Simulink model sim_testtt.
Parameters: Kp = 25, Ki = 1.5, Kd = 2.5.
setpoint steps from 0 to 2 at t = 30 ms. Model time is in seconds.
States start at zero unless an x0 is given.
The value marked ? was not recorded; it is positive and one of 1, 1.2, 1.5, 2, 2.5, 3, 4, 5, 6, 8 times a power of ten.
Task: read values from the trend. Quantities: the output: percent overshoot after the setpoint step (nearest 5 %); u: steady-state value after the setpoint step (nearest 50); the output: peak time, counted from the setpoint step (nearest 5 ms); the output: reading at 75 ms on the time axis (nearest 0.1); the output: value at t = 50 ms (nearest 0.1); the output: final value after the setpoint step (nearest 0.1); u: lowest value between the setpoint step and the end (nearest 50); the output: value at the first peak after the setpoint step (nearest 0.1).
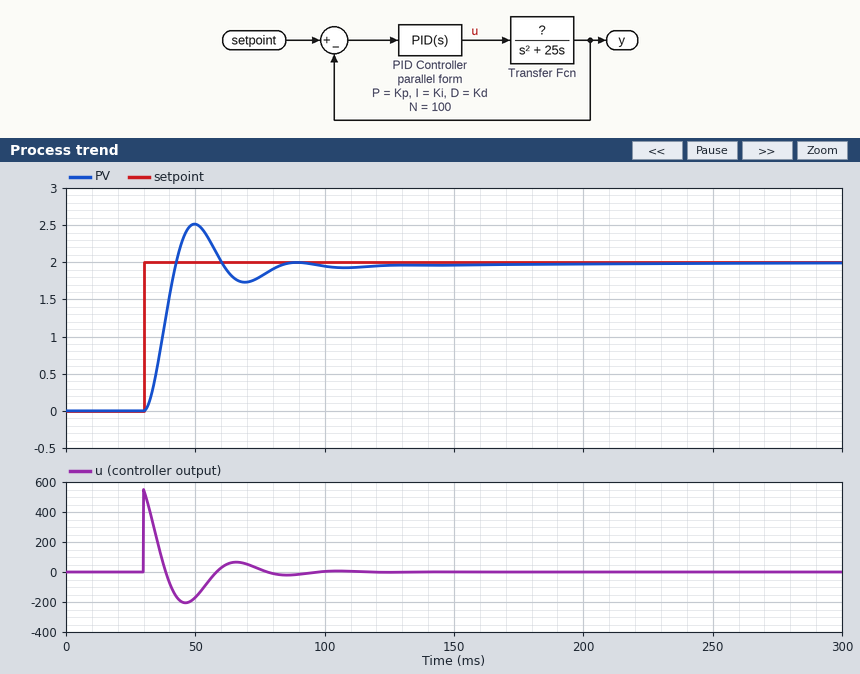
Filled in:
25 %
0
20 ms
1.8
2.5
2.0
-200
2.5
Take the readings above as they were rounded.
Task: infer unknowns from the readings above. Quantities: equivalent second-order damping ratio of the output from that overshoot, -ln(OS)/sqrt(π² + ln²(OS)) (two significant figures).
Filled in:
0.40
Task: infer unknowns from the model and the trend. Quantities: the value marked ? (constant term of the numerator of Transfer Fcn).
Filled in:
100
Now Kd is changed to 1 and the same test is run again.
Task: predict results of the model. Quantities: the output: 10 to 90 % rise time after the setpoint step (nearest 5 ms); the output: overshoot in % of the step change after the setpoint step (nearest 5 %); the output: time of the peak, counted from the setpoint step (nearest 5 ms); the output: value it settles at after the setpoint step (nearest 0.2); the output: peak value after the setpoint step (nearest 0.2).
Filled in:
15 ms
15 %
30 ms
2.0
2.4
